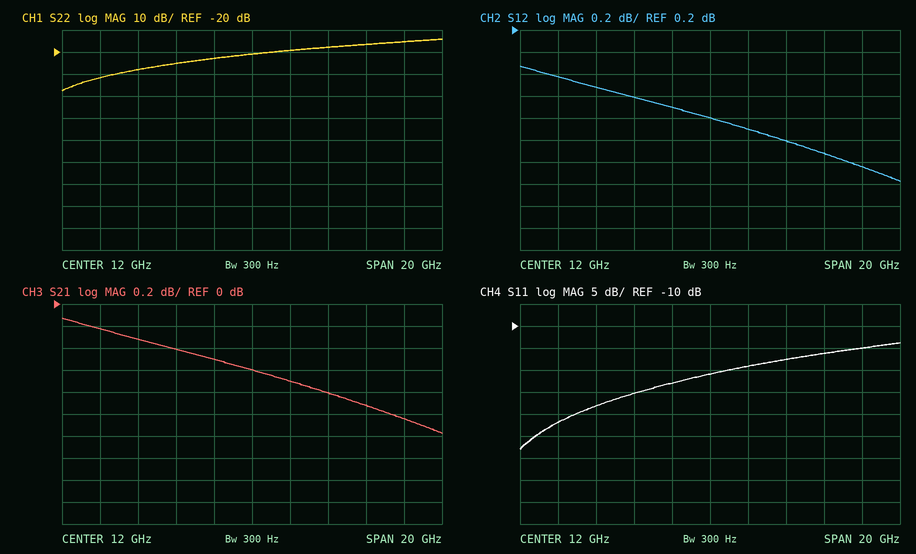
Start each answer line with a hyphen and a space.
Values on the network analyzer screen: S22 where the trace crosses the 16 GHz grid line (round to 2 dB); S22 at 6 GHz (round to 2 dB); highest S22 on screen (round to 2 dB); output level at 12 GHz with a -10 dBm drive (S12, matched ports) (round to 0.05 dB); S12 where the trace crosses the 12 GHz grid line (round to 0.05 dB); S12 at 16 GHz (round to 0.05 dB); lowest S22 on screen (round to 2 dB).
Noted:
- -18 dB
- -28 dB
- -14 dB
- -10.60 dBm
- -0.60 dB
- -0.80 dB
- -38 dB
